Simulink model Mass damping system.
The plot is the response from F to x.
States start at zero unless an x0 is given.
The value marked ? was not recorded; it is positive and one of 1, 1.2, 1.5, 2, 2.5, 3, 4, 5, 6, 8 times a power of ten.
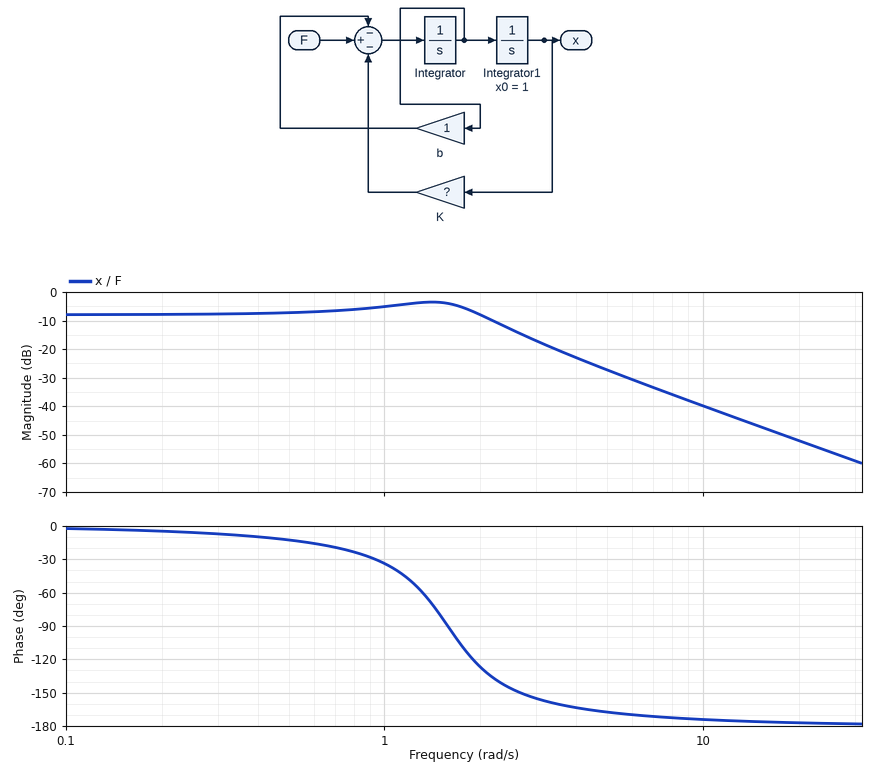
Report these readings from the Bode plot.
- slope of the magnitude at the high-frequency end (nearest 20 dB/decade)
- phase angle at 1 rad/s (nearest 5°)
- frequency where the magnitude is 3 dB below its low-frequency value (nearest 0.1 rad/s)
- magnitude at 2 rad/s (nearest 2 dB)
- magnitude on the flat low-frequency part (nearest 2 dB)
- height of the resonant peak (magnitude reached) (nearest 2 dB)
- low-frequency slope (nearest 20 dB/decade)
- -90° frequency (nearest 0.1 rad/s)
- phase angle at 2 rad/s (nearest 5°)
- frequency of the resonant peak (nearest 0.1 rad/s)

-40 dB/decade
-35°
2.3 rad/s
-8 dB
-8 dB
-4 dB
0 dB/decade
1.6 rad/s
-125°
1.4 rad/s
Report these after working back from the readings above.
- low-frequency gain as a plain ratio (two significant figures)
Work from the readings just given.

0.40
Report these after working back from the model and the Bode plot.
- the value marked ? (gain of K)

2.5
